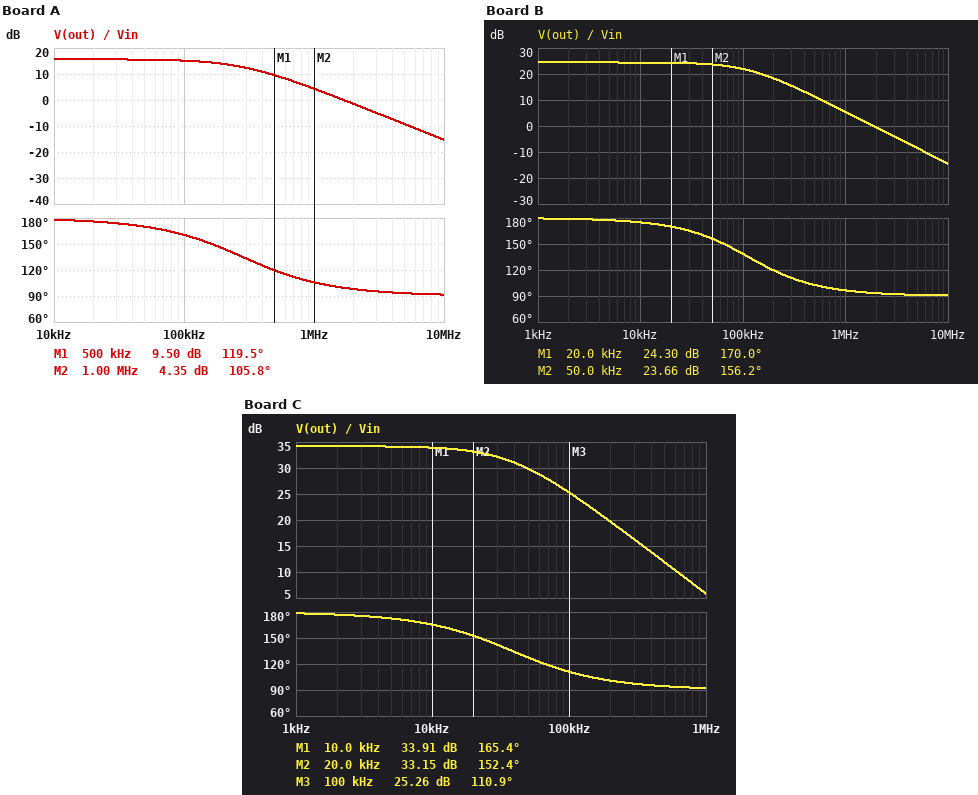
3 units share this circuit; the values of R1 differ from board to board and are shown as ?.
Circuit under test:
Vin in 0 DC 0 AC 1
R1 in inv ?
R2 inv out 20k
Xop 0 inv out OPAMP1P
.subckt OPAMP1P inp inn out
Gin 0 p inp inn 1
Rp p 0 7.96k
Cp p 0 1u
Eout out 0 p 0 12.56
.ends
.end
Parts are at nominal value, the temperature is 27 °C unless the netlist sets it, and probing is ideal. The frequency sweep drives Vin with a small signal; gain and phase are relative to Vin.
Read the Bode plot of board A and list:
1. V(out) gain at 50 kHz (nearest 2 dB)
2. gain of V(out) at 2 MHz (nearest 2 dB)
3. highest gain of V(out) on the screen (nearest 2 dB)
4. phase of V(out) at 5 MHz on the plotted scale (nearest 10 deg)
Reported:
16 dB
-2 dB
16 dB
90 deg
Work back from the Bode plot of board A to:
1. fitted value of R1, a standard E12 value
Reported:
3.3 kΩ
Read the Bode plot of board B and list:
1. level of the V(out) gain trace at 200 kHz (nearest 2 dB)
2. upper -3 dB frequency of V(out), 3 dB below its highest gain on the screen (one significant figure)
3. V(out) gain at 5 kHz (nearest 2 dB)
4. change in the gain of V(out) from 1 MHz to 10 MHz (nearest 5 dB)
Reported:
18 dB
100 kHz
24 dB
-20 dB
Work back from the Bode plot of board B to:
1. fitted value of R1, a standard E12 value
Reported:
1.2 kΩ
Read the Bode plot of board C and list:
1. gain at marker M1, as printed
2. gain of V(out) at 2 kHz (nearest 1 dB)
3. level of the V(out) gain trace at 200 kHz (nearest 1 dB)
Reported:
33.91 dB
34 dB
20 dB
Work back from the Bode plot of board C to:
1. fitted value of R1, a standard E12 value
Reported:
390 Ω
